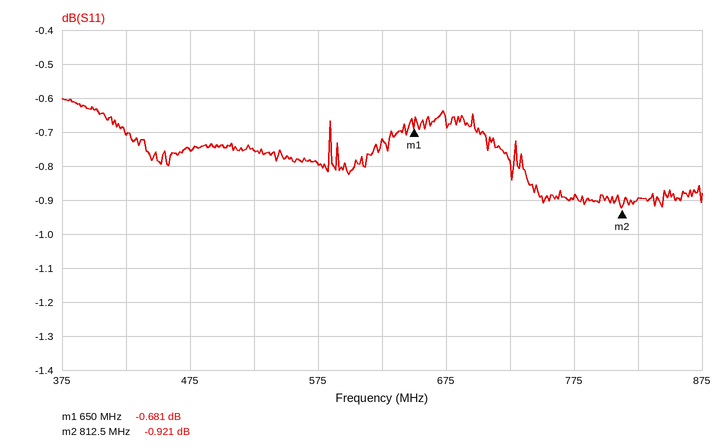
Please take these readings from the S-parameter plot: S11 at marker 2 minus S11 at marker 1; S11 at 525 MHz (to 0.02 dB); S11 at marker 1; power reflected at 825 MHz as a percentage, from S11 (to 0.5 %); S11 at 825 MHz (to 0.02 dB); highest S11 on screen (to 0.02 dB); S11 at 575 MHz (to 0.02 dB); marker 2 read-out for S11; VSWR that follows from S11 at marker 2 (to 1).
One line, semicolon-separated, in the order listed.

-0.240 dB; -0.76 dB; -0.681 dB; 81.5 %; -0.90 dB; -0.60 dB; -0.80 dB; -0.921 dB; 19
